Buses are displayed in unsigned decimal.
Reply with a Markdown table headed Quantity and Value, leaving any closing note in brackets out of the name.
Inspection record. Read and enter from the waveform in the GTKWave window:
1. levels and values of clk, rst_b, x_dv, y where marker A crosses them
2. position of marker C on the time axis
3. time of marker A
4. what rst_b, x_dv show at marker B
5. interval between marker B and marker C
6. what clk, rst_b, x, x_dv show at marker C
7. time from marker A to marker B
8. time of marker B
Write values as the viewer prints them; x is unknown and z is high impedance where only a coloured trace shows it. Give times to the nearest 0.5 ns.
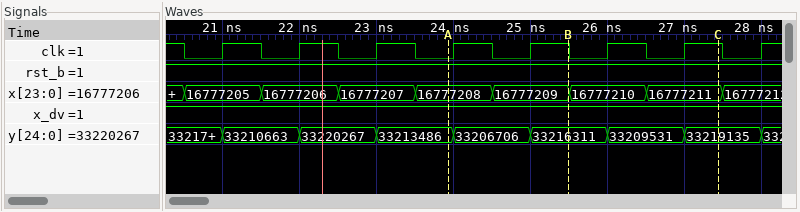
| Quantity | Value |
|---|---|
| levels and values of clk, rst_b, x_dv, y where marker A crosses them | clk=0, rst_b=1, x_dv=1, y=33213486 |
| position of marker C on the time axis | 27.5 ns |
| time of marker A | 24 ns |
| what rst_b, x_dv show at marker B | rst_b=1, x_dv=1 |
| interval between marker B and marker C | 2 ns |
| what clk, rst_b, x, x_dv show at marker C | clk=1, rst_b=1, x=16777211, x_dv=1 |
| time from marker A to marker B | 1.5 ns |
| time of marker B | 25.5 ns |
